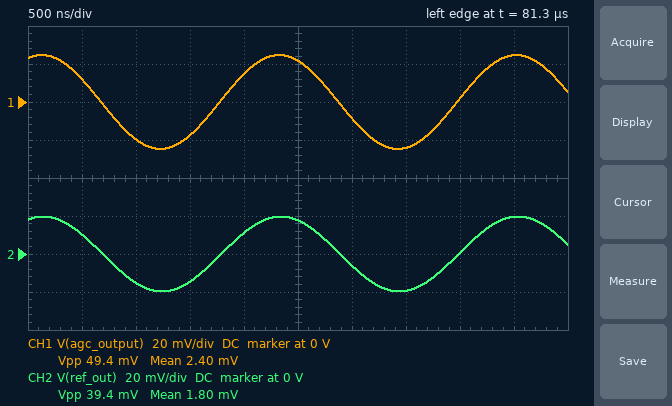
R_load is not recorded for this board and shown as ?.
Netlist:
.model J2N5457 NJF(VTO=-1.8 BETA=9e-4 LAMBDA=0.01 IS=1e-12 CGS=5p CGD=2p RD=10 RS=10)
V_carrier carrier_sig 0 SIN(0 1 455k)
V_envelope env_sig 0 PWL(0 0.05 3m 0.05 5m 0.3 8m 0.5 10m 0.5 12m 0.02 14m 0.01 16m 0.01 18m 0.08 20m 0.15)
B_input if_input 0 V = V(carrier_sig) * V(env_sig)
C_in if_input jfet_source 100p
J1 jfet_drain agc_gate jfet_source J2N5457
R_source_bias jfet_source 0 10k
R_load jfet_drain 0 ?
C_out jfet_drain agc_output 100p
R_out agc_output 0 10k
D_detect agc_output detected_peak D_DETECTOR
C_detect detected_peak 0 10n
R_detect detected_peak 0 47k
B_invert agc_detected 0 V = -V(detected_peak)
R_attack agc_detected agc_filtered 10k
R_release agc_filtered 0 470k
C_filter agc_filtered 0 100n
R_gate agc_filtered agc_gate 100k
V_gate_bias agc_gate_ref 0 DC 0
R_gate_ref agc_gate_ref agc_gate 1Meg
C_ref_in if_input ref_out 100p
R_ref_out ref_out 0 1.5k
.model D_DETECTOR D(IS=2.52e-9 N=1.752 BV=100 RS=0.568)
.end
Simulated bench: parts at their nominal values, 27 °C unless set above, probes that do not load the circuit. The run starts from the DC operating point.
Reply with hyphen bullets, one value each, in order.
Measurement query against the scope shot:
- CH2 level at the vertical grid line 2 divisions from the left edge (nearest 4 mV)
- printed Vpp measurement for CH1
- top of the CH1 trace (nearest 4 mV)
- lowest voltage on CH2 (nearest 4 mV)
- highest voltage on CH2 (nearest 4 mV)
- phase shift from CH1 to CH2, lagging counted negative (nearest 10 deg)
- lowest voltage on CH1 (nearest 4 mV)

- -16 mV
- 49.4 mV
- 24 mV
- -20 mV
- 20 mV
- 0 deg
- -24 mV
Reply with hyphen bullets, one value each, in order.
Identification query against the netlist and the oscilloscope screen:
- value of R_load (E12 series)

- 4.7 kΩ
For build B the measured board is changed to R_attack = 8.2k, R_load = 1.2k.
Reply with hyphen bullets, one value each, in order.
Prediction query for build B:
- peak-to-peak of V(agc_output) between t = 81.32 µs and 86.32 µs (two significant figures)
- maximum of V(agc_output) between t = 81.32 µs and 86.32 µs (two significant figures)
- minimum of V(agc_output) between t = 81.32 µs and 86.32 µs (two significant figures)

- 24 mV
- 12 mV
- -12 mV
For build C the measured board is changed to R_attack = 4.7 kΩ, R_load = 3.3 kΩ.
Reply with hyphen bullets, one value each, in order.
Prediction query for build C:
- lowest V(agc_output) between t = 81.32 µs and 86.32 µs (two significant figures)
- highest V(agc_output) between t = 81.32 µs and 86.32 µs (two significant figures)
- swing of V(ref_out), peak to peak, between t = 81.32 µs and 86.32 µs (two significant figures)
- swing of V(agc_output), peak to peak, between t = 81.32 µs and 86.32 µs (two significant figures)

- -22 mV
- 22 mV
- 39 mV
- 43 mV
